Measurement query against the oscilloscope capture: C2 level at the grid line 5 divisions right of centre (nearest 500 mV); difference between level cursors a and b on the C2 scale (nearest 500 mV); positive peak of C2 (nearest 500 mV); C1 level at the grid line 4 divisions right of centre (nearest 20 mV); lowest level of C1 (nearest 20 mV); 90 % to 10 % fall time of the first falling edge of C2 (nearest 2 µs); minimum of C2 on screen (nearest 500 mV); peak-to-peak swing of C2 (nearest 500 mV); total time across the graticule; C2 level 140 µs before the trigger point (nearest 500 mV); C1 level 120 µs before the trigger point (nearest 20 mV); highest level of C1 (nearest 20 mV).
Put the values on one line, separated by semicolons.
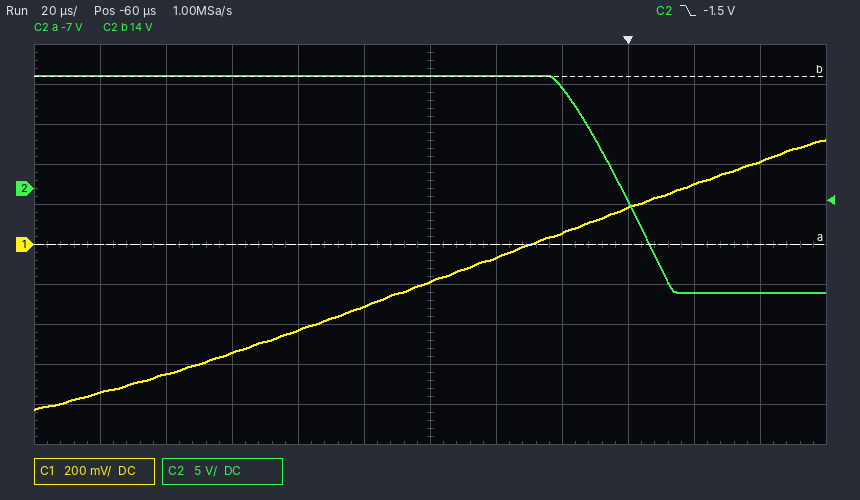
-13.0 V; 21.0 V; 14.0 V; 300 mV; -820 mV; 28 µs; -13.0 V; 27.0 V; 240 µs; 14.0 V; -540 mV; 520 mV
